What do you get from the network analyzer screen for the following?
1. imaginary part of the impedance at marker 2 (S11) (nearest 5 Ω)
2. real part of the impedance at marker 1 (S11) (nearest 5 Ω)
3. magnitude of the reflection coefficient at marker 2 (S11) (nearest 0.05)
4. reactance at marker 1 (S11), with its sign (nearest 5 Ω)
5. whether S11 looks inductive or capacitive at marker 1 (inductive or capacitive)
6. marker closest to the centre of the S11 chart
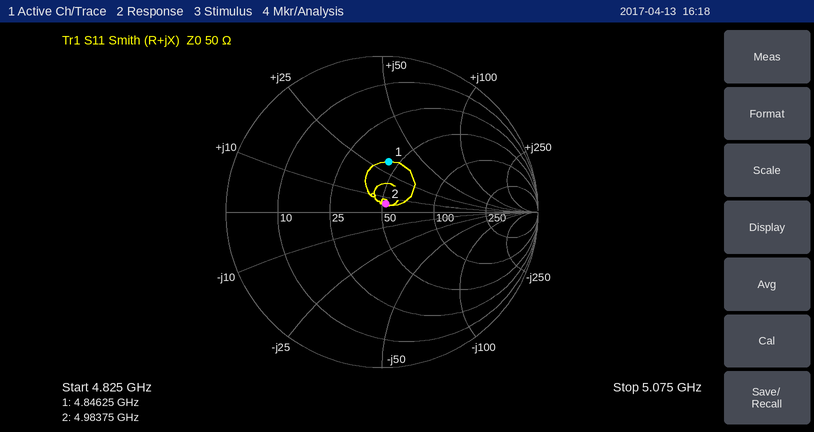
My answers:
+5 Ω
45 Ω
0.05
+30 Ω
inductive
marker 2
